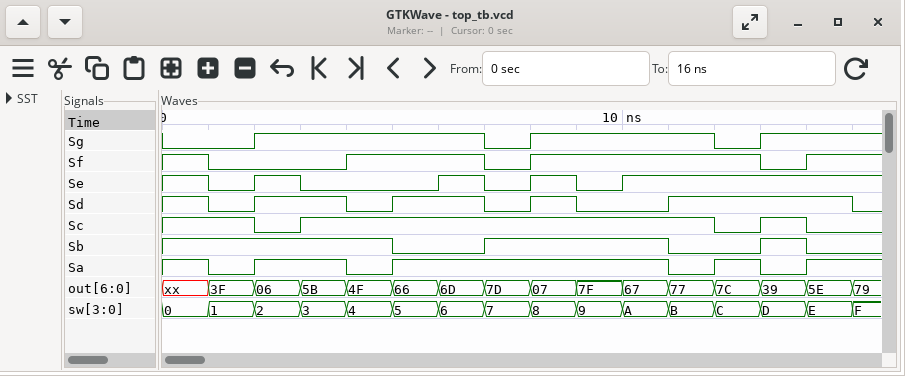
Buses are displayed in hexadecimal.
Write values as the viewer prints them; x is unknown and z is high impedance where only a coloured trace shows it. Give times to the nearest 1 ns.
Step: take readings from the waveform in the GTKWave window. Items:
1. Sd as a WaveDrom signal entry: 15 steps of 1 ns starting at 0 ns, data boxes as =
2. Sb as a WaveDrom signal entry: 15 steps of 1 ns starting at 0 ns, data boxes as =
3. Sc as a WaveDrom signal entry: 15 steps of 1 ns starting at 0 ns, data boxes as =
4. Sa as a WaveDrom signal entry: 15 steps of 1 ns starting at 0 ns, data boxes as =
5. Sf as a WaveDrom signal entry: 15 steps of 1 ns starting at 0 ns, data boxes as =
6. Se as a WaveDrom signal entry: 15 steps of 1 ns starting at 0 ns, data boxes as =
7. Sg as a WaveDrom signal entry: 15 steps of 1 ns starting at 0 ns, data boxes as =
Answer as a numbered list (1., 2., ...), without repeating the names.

1. {name: 'Sd', wave: '101.01.010.1...'}
2. {name: 'Sb', wave: '1....0.1...0.10'}
3. {name: 'Sc', wave: '1.01........010'}
4. {name: 'Sa', wave: '101.01.....0101'}
5. {name: 'Sf', wave: '10..1..01....01'}
6. {name: 'Se', wave: '1010..10101....'}
7. {name: 'Sg', wave: '0.1....01...01.'}
